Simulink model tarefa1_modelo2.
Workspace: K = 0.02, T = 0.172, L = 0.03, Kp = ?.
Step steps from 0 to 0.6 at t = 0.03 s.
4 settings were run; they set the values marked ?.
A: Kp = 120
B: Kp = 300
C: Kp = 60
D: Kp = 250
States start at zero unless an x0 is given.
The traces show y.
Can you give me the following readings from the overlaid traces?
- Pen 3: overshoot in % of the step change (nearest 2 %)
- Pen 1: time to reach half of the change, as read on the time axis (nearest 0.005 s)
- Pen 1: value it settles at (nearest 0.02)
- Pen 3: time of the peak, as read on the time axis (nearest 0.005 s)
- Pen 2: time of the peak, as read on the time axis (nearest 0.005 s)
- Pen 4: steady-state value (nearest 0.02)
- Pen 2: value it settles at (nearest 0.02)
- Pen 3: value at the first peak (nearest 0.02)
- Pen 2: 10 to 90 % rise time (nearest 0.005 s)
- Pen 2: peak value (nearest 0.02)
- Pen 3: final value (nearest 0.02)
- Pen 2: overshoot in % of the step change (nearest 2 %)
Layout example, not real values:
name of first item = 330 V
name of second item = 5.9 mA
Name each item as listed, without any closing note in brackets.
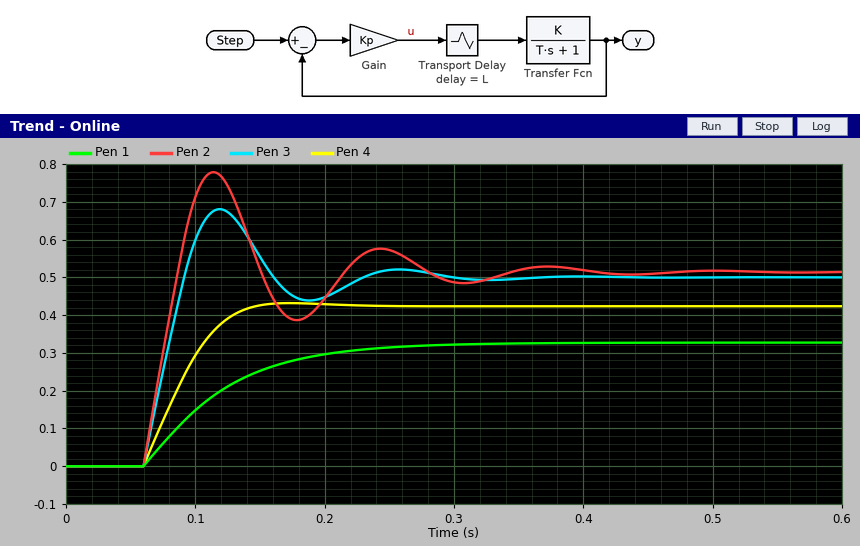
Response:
Pen 3: overshoot in % of the step change = 36 %
Pen 1: time to reach half of the change, as read on the time axis = 0.105 s
Pen 1: value it settles at = 0.32
Pen 3: time of the peak, as read on the time axis = 0.120 s
Pen 2: time of the peak, as read on the time axis = 0.115 s
Pen 4: steady-state value = 0.42
Pen 2: value it settles at = 0.52
Pen 3: value at the first peak = 0.68
Pen 2: 10 to 90 % rise time = 0.020 s
Pen 2: peak value = 0.78
Pen 3: final value = 0.50
Pen 2: overshoot in % of the step change = 52 %
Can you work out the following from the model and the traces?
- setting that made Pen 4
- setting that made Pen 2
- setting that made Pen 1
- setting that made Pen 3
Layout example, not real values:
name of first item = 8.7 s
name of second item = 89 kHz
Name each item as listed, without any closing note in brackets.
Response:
setting that made Pen 4 = A
setting that made Pen 2 = B
setting that made Pen 1 = C
setting that made Pen 3 = D
